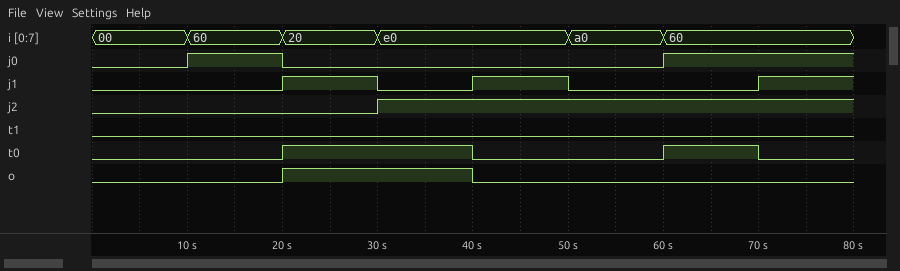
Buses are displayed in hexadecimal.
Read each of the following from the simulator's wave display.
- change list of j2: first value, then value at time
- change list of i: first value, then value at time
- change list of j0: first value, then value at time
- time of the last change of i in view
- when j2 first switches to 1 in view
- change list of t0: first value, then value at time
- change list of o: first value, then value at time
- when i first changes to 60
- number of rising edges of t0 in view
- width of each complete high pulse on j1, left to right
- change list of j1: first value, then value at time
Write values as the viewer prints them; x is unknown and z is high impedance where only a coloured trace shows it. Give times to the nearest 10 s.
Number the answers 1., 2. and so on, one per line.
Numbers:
1. 0, 1 at 30 s
2. 00, 60 at 10 s, 20 at 20 s, e0 at 30 s, a0 at 50 s, 60 at 60 s
3. 0, 1 at 10 s, 0 at 20 s, 1 at 60 s
4. 60 s
5. 30 s
6. 0, 1 at 20 s, 0 at 40 s, 1 at 60 s, 0 at 70 s
7. 0, 1 at 20 s, 0 at 40 s
8. 10 s
9. 2
10. 10 s, 10 s
11. 0, 1 at 20 s, 0 at 30 s, 1 at 40 s, 0 at 50 s, 1 at 70 s
